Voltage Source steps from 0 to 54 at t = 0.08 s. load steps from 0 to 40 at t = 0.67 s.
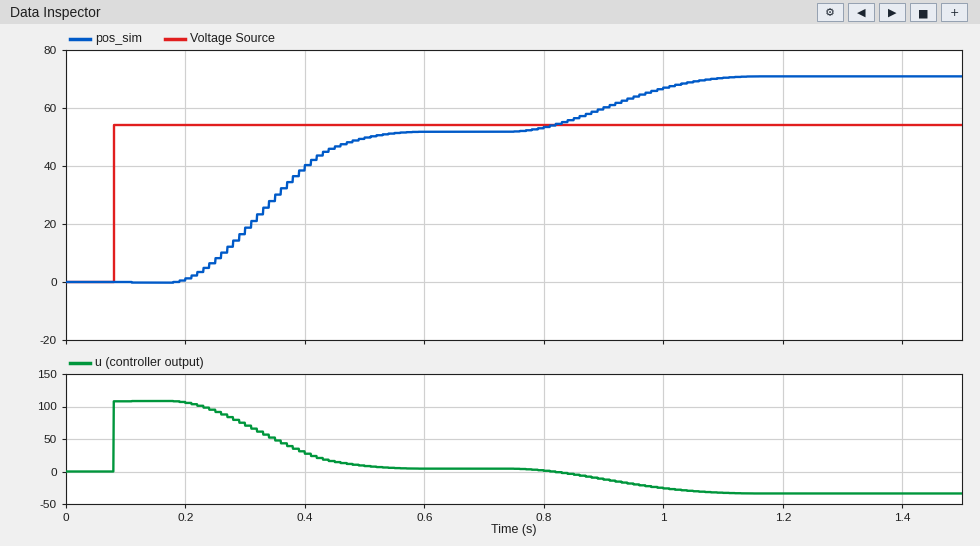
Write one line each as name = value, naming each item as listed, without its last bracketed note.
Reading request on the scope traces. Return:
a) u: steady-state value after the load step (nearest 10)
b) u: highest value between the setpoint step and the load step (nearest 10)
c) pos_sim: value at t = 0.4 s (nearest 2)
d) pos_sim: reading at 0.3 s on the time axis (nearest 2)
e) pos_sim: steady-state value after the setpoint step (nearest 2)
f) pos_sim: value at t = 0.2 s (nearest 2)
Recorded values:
u: steady-state value after the load step = -30
u: highest value between the setpoint step and the load step = 110
pos_sim: value at t = 0.4 s = 40
pos_sim: reading at 0.3 s on the time axis = 18
pos_sim: steady-state value after the setpoint step = 52
pos_sim: value at t = 0.2 s = 2
